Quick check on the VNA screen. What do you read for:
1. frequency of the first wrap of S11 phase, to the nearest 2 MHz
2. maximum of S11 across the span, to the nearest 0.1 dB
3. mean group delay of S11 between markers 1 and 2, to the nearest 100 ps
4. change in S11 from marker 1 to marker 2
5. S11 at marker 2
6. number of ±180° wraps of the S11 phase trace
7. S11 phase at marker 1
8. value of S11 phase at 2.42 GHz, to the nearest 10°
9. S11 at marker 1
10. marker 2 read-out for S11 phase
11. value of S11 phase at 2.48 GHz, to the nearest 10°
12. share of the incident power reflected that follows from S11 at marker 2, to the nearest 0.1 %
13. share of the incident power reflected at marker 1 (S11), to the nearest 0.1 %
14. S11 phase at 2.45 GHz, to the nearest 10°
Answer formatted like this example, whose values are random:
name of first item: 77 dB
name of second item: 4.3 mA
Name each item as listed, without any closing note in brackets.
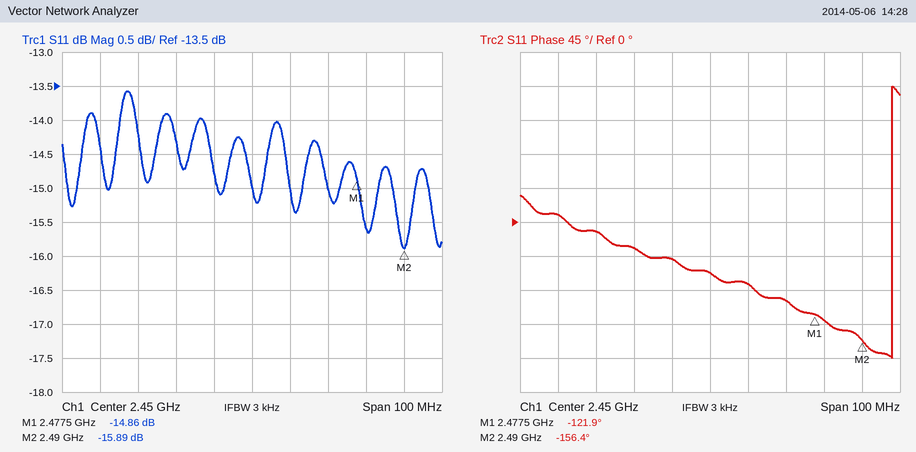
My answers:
frequency of the first wrap of S11 phase, to the nearest 2 MHz: 2.498 GHz
maximum of S11 across the span, to the nearest 0.1 dB: -13.6 dB
mean group delay of S11 between markers 1 and 2, to the nearest 100 ps: 7.7 ns
change in S11 from marker 1 to marker 2: -1.03 dB
S11 at marker 2: -15.89 dB
number of ±180° wraps of the S11 phase trace: 1
S11 phase at marker 1: -121.9°
value of S11 phase at 2.42 GHz, to the nearest 10°: -10°
S11 at marker 1: -14.86 dB
marker 2 read-out for S11 phase: -156.4°
value of S11 phase at 2.48 GHz, to the nearest 10°: -130°
share of the incident power reflected that follows from S11 at marker 2, to the nearest 0.1 %: 2.6 %
share of the incident power reflected at marker 1 (S11), to the nearest 0.1 %: 3.3 %
S11 phase at 2.45 GHz, to the nearest 10°: -70°
